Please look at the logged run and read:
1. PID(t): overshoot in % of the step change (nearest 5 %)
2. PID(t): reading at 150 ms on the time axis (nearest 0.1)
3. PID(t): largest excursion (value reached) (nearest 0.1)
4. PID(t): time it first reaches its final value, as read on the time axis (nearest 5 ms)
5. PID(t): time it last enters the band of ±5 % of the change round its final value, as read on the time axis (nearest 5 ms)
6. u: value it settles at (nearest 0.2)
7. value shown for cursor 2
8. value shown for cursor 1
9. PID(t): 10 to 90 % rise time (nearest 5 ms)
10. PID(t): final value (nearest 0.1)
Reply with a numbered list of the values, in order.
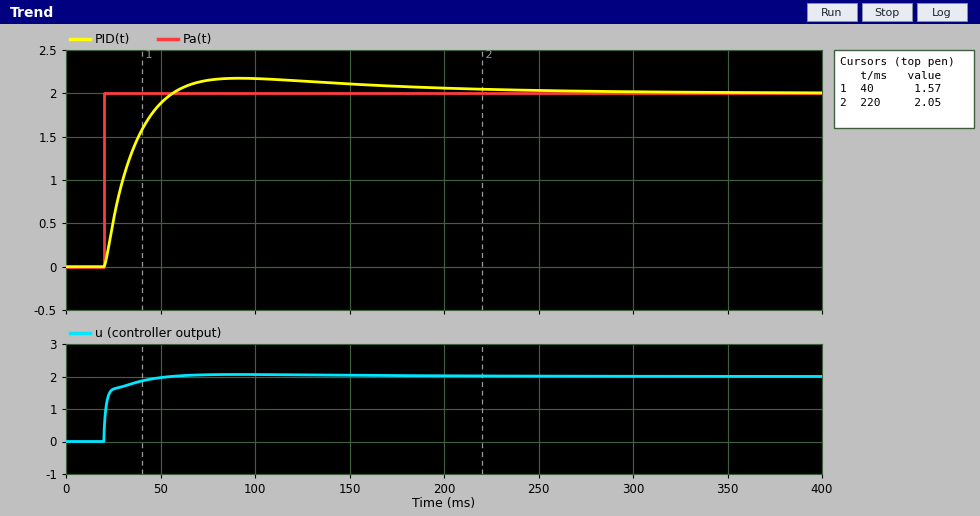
1. 10 %
2. 2.1
3. 2.2
4. 55 ms
5. 155 ms
6. 2.0
7. 2.05
8. 1.57
9. 25 ms
10. 2.0
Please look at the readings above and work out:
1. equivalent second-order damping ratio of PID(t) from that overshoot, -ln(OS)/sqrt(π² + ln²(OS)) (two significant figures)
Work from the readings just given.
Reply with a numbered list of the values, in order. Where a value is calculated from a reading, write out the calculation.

1. ln(0.1) = -2.303; 2.303 / sqrt(9.870 + 5.302) = 0.59
